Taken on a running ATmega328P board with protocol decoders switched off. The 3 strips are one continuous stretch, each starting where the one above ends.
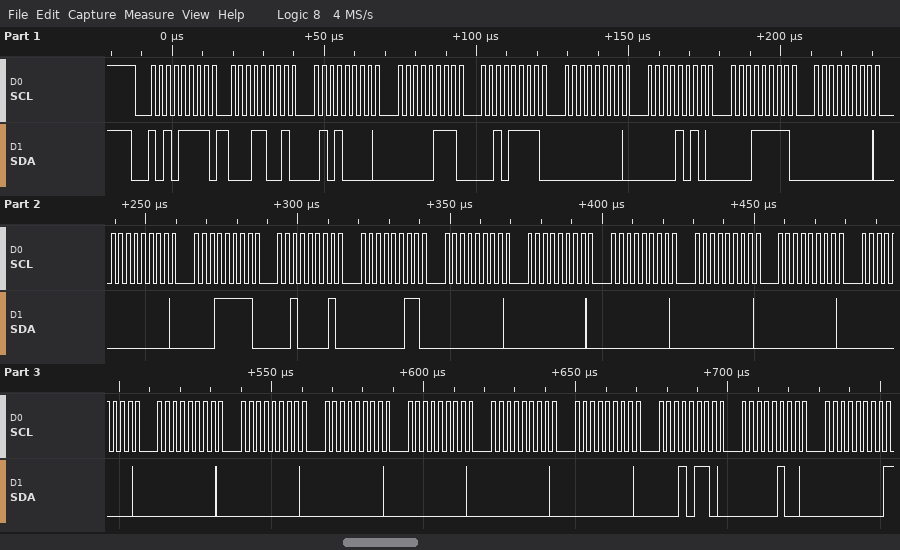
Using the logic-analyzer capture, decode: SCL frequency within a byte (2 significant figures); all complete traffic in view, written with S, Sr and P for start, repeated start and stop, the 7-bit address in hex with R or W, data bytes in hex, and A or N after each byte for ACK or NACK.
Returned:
400 kHz
S 57R A 19 A 50 A 07 A 2F A 00 A 0A A 1F A 00 A 00 A 1F A 21 A 03 A 00 A 00 A 00 A 00 A 00 A 00 A 00 A 00 A 00 A 00 A 00 A 00 A 16 A 04 A 00 N
